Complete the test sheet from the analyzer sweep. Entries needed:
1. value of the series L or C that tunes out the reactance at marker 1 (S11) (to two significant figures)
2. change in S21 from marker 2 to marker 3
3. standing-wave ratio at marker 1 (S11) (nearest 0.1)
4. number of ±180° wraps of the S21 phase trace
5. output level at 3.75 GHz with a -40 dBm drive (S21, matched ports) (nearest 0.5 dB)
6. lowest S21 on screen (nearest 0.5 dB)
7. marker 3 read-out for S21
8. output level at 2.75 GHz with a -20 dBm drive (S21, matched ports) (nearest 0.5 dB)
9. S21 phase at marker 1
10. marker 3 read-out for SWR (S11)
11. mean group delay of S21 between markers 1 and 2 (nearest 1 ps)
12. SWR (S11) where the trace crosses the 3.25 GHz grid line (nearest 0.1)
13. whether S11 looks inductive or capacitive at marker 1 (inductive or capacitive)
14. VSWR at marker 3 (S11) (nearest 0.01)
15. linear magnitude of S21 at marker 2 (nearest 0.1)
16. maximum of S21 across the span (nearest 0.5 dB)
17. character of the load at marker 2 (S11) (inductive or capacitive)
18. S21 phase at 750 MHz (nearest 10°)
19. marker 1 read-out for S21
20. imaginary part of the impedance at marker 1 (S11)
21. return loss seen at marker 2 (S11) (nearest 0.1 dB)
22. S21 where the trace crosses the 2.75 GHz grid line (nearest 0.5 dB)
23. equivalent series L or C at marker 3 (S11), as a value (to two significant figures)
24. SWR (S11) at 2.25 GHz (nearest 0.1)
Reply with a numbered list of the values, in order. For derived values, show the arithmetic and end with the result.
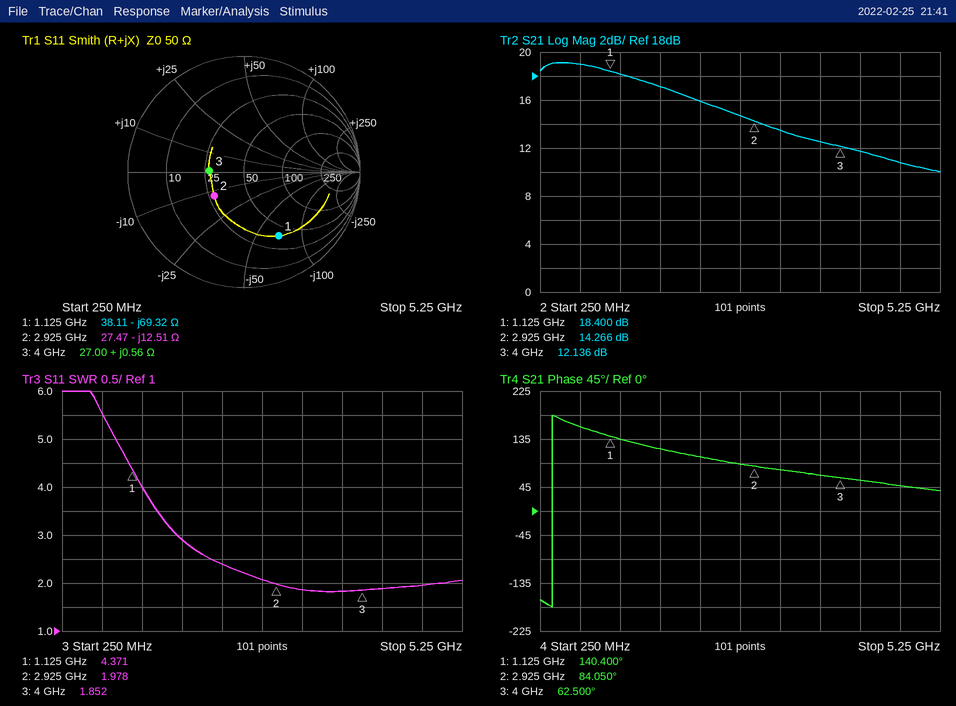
1. L = 69.32 Ω/(2π × 1.125 GHz) ≈ 9.8 nH
2. 12.136 − (14.266) = -2.130 dB
3. 4.4
4. 1
5. -40 dBm + (12.5 dB) = -27.5 dBm
6. 10.0 dB
7. 12.136 dB
8. -20 dBm + (14.5 dB) = -5.5 dBm
9. 140.400°
10. 1.852
11. −(84.05° − (140.4°))/(360° × 1.8 GHz) ≈ 87 ps
12. 1.9
13. capacitive
14. 1.85
15. 10^(14.266/20) ≈ 5.2
16. 19.0 dB
17. capacitive
18. 160°
19. 18.400 dB
20. -69.32 Ω
21. 9.7 dB
22. 14.5 dB
23. L = 0.56 Ω/(2π × 4 GHz) ≈ 22 pH
24. 2.4
